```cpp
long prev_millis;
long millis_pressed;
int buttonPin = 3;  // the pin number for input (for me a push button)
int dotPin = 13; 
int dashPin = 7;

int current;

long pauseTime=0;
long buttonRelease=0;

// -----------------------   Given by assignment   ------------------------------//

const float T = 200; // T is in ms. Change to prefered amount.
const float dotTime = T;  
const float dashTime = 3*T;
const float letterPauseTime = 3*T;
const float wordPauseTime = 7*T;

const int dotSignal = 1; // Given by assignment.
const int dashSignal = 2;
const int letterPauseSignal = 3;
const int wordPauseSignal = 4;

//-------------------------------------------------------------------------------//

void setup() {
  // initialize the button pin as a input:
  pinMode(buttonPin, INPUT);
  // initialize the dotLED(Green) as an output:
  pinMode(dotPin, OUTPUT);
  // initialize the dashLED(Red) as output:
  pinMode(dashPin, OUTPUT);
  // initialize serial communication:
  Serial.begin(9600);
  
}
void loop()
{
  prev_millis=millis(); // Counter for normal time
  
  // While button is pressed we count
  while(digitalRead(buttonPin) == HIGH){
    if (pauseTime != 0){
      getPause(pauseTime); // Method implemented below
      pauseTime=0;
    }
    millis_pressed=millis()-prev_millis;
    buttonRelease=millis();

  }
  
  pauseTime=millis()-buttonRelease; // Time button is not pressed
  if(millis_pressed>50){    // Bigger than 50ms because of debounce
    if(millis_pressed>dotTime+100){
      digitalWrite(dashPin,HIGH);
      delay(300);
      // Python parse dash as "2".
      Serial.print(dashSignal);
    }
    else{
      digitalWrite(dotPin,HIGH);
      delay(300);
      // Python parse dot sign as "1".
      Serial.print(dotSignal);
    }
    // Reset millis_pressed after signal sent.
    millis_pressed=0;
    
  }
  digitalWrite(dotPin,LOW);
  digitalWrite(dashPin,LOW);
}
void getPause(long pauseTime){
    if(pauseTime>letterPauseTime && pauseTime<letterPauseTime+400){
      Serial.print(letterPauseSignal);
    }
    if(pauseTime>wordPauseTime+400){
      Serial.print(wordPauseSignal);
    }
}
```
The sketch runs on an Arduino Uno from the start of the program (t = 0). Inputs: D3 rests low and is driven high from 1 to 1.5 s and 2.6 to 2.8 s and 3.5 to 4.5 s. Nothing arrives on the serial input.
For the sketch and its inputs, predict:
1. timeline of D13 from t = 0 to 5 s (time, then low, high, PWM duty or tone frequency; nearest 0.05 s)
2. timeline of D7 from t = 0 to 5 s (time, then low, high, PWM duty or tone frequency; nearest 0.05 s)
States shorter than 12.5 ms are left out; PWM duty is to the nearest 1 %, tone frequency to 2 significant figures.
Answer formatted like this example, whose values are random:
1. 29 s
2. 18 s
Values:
1. 0 s low; 2.8 s high; 3.1 s low
2. 0 s low; 1.5 s high; 1.8 s low; 4.5 s high; 4.8 s low
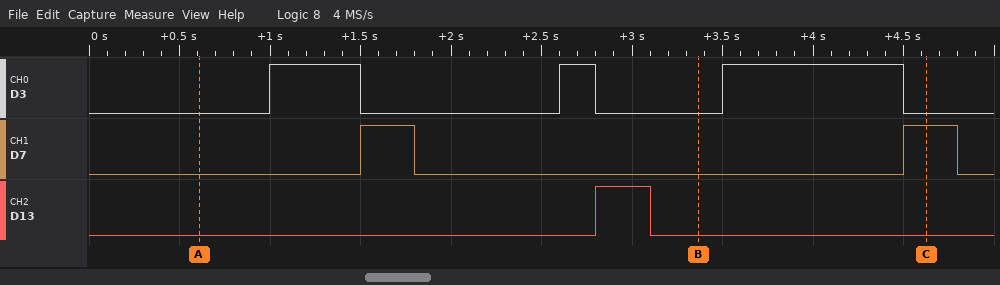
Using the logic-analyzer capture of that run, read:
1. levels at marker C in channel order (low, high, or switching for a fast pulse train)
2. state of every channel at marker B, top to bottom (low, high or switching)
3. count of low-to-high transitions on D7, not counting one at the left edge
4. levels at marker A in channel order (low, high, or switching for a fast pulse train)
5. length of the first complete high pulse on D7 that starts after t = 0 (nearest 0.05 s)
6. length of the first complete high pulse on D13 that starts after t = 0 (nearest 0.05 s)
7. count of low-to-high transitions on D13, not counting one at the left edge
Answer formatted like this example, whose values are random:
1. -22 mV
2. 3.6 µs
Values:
1. D3 low, D7 high, D13 low
2. D3 low, D7 low, D13 low
3. 2
4. D3 low, D7 low, D13 low
5. 0.30 s
6. 0.30 s
7. 1
